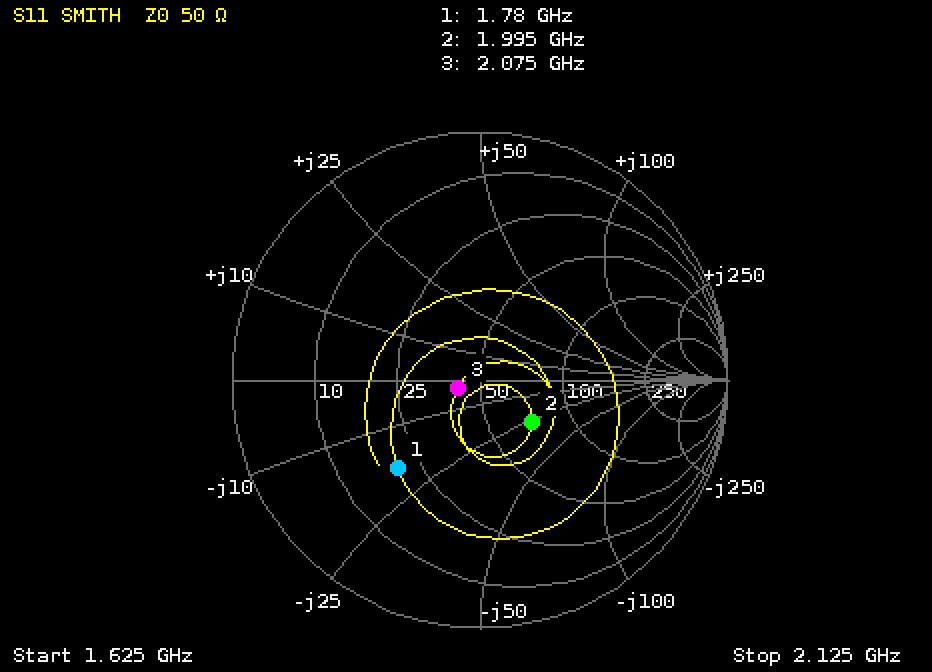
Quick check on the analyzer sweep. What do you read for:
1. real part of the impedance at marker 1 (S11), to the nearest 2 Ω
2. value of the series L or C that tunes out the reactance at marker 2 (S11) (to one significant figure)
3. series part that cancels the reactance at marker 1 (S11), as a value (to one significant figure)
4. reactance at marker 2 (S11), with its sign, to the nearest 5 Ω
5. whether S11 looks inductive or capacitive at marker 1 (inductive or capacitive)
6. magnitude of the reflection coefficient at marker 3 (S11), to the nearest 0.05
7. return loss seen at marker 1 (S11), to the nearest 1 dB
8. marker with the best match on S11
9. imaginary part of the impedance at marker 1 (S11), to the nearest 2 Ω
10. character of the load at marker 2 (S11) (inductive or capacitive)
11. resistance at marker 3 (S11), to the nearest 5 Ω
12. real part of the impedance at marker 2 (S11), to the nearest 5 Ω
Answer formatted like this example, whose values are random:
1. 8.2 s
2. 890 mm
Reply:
1. 20 Ω
2. 2 nH
3. 2 nH
4. -25 Ω
5. capacitive
6. 0.10
7. 6 dB
8. marker 3
9. -18 Ω
10. capacitive
11. 40 Ω
12. 70 Ω
